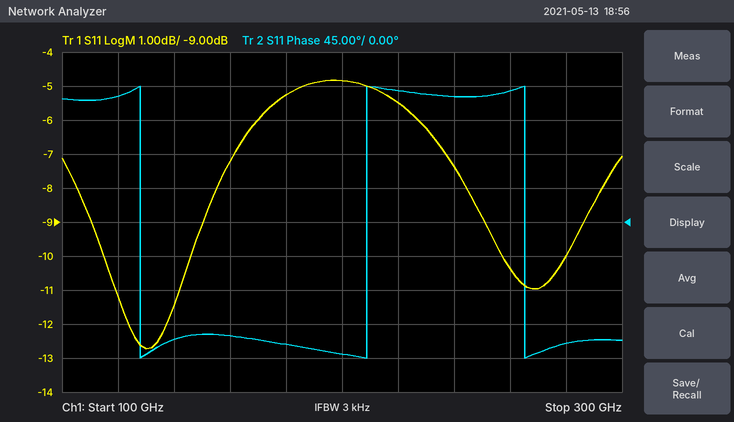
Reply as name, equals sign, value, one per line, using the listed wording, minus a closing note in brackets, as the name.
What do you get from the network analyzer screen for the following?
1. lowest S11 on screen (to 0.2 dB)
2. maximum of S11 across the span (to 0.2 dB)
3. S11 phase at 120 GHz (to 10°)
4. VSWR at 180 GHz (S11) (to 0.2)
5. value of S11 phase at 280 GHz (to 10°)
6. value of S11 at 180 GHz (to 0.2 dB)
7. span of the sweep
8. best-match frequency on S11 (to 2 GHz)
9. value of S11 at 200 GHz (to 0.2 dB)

lowest S11 on screen = -12.8 dB
maximum of S11 across the span = -4.8 dB
S11 phase at 120 GHz = 170°
VSWR at 180 GHz (S11) = 3.4
value of S11 phase at 280 GHz = -160°
value of S11 at 180 GHz = -5.2 dB
span of the sweep = 200 GHz
best-match frequency on S11 = 130 GHz
value of S11 at 200 GHz = -4.8 dB
